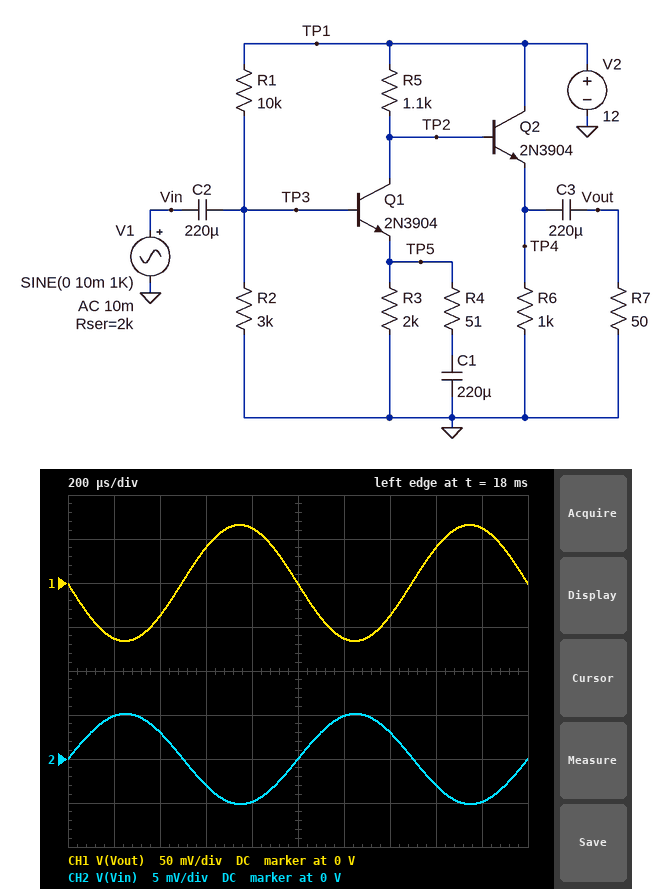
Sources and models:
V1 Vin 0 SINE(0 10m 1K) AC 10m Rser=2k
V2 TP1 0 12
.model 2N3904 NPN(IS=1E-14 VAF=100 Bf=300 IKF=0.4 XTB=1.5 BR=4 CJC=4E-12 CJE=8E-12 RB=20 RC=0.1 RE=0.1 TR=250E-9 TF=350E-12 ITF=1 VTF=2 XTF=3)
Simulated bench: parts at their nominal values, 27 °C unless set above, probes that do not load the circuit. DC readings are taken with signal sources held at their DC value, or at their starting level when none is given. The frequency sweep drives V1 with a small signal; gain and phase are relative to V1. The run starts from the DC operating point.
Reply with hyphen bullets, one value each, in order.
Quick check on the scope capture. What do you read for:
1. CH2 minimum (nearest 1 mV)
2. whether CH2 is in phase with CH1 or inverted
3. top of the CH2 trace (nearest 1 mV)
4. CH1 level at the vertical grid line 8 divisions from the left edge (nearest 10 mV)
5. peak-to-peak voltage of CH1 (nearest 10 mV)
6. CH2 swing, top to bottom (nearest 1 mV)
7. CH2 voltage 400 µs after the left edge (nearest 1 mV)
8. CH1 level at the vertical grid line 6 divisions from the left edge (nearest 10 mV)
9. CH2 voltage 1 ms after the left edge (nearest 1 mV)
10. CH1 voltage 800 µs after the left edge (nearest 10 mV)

- -5 mV
- inverted
- 5 mV
- 40 mV
- 130 mV
- 10 mV
- 3 mV
- -60 mV
- 0 V
- 60 mV
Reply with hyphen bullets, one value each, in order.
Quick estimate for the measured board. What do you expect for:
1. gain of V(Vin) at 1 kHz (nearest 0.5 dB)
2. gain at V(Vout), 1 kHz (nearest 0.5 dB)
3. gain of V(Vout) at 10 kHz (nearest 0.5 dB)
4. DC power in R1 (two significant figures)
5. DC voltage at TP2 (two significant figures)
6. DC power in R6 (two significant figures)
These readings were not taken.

- -6.0 dB
- 16.5 dB
- 16.5 dB
- 8.5 mW
- 11 V
- 100 mW
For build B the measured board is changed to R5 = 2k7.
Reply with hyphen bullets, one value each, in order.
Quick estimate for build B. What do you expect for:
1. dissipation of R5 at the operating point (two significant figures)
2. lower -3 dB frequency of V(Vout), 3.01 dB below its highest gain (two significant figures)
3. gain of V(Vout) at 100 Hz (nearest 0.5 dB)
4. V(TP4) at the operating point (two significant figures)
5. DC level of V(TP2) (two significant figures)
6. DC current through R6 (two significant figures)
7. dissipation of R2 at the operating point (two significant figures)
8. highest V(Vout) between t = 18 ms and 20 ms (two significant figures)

- 3.1 mW
- 16 Hz
- 23.0 dB
- 8.4 V
- 9.1 V
- 8.4 mA
- 2.5 mW
- 150 mV
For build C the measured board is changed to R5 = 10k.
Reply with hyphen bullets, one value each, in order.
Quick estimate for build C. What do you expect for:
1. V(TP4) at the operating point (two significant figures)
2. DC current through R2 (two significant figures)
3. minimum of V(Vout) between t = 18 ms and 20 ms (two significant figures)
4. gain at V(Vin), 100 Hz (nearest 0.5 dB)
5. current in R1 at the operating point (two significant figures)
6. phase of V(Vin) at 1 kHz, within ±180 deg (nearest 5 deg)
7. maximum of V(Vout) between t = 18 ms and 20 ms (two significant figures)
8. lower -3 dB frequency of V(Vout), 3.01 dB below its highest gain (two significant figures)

- 1.4 V
- 900 µA
- -2.1 mV
- -22.0 dB
- 930 µA
- 0 deg
- 2.4 mV
- 11 Hz
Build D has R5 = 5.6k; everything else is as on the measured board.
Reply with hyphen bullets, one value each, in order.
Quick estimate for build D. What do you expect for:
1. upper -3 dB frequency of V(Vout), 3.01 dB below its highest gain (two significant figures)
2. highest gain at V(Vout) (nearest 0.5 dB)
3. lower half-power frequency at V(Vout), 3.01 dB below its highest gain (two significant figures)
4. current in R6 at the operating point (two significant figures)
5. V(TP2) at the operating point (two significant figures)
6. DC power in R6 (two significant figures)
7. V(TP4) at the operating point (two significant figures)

- 840 kHz
- 28.0 dB
- 15 Hz
- 5.3 mA
- 6.0 V
- 28 mW
- 5.3 V
